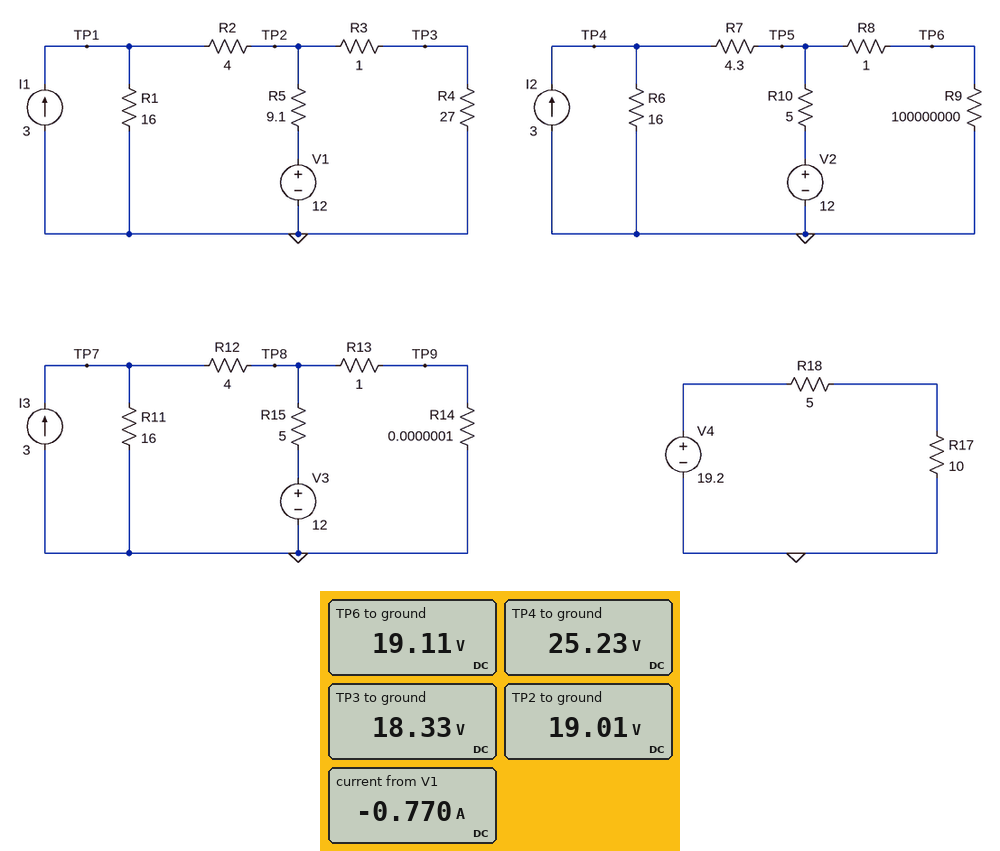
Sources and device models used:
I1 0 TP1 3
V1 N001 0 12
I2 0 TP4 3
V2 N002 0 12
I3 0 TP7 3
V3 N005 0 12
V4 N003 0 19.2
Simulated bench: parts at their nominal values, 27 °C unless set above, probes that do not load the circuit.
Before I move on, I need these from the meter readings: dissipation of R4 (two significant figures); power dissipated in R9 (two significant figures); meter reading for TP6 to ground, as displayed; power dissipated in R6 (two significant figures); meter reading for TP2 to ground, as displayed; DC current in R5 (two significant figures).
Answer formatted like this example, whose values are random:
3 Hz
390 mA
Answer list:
12 W
3.7 µW
19.11 V
40 W
19.01 V
770 mA
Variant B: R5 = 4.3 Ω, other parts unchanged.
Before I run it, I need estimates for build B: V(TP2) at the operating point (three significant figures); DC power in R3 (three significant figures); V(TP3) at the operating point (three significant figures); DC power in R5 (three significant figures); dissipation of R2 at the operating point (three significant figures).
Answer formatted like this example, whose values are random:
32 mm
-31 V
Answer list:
16.3 V
339 mW
15.7 V
4.32 W
10.0 W
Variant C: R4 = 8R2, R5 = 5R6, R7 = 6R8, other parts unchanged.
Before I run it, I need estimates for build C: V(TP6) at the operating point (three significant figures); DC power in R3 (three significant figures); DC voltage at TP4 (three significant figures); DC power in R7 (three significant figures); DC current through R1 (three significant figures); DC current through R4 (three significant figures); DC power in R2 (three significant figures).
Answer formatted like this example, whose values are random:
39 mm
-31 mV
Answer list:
18.5 V
2.14 W
27.3 V
11.4 W
1.27 A
1.46 A
11.9 W
